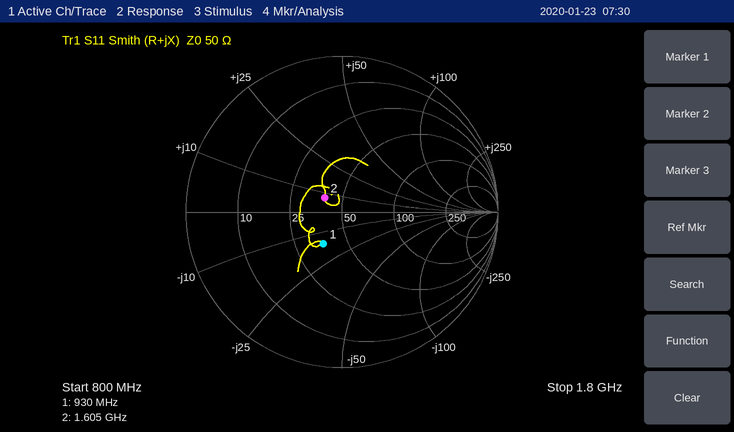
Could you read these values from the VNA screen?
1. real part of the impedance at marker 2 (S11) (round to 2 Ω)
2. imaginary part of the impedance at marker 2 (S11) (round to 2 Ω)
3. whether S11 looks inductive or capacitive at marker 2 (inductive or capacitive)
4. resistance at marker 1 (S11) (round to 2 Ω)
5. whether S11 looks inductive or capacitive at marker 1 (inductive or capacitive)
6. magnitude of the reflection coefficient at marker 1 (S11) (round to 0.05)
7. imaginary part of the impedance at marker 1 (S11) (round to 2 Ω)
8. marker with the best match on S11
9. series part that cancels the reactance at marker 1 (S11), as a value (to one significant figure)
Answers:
40 Ω
+8 Ω
inductive
36 Ω
capacitive
0.25
-16 Ω
marker 2
3 nH
